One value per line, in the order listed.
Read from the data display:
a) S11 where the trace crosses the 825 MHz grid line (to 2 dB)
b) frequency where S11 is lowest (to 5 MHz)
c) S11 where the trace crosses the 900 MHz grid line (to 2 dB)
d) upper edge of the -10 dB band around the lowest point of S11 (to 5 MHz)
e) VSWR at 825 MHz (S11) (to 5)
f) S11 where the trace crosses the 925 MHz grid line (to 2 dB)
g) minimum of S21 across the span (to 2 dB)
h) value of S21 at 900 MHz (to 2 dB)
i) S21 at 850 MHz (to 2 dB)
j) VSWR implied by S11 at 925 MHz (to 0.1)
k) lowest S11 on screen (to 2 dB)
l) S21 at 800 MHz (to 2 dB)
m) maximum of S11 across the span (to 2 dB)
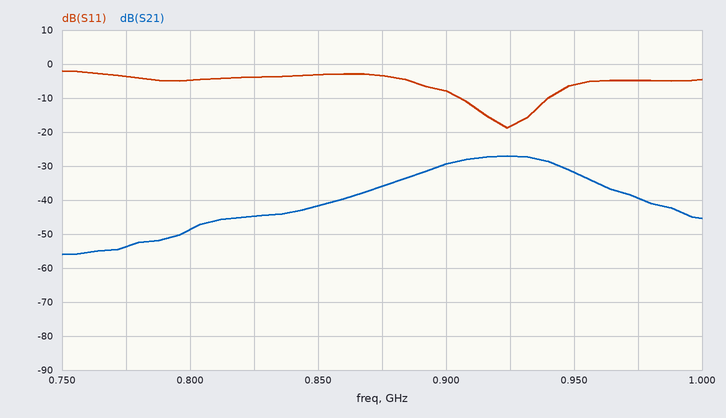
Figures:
-4 dB
925 MHz
-8 dB
940 MHz
5
-18 dB
-56 dB
-30 dB
-42 dB
1.3
-18 dB
-48 dB
-2 dB
